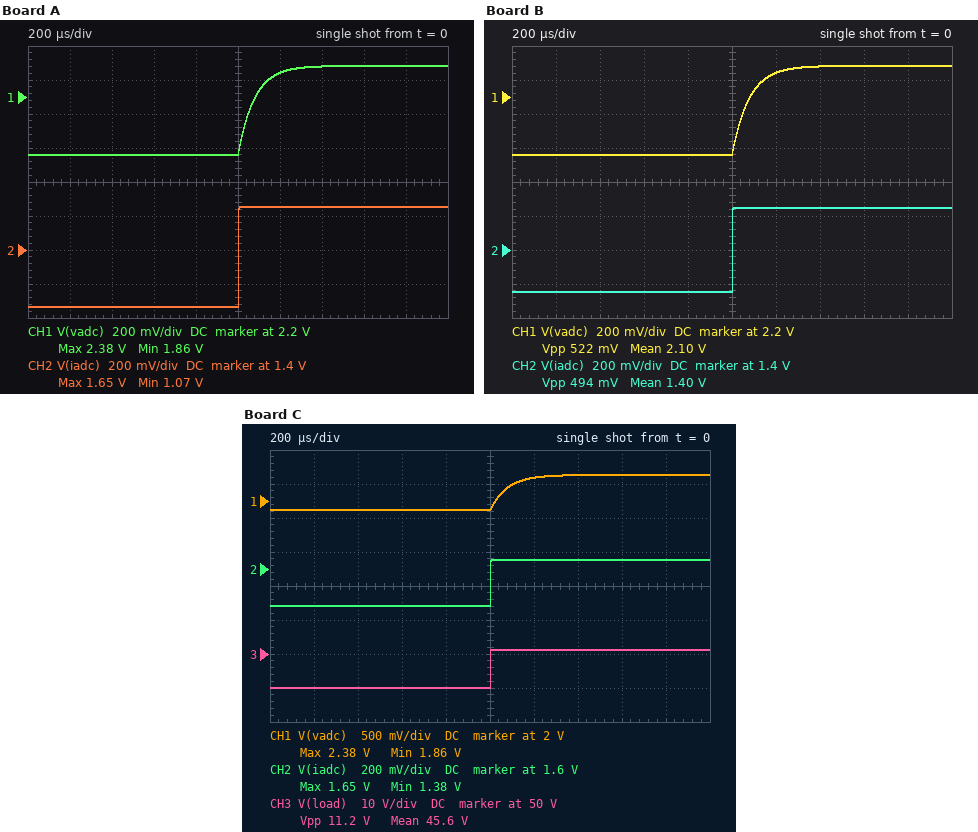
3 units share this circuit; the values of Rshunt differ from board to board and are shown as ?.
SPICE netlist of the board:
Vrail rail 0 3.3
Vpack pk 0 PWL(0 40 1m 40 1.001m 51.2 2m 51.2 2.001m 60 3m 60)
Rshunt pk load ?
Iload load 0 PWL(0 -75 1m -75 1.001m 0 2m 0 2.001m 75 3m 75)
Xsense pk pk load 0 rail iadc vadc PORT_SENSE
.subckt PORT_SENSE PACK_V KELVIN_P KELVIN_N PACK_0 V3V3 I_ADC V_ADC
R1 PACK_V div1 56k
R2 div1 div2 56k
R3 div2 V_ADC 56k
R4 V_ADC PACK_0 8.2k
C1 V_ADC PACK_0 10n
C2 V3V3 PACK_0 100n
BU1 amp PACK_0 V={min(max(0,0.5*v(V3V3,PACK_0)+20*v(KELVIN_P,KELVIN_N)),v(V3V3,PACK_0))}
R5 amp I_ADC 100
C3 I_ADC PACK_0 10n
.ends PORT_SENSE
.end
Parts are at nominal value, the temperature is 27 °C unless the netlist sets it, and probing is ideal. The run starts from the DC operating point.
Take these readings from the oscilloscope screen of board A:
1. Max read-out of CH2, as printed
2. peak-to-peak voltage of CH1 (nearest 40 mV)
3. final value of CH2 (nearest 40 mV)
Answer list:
1.65 V
520 mV
1.64 V
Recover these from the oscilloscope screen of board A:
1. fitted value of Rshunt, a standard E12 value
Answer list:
390 µΩ
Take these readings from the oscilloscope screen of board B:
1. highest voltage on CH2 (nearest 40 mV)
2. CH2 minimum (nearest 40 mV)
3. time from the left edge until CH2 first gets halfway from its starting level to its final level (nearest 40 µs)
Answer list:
1.64 V
1.16 V
1.00 ms
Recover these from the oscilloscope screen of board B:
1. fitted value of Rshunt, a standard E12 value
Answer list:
330 µΩ
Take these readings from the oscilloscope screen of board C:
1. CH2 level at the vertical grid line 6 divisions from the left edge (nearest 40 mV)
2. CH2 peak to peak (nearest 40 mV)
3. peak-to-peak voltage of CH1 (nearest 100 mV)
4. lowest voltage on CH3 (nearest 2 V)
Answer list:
1.64 V
280 mV
500 mV
40 V
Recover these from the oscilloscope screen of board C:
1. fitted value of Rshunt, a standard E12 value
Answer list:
180 µΩ
